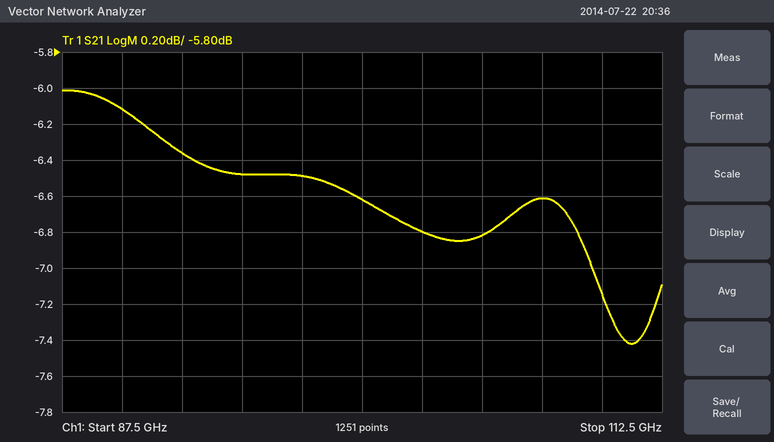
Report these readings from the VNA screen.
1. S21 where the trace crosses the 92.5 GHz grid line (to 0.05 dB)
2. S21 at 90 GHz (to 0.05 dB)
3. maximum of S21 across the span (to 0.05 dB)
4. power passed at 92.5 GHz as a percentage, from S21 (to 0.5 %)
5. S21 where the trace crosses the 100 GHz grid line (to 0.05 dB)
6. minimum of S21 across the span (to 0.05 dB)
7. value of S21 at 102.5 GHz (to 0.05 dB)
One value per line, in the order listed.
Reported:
-6.35 dB
-6.10 dB
-6.00 dB
23.0 %
-6.60 dB
-7.40 dB
-6.80 dB
